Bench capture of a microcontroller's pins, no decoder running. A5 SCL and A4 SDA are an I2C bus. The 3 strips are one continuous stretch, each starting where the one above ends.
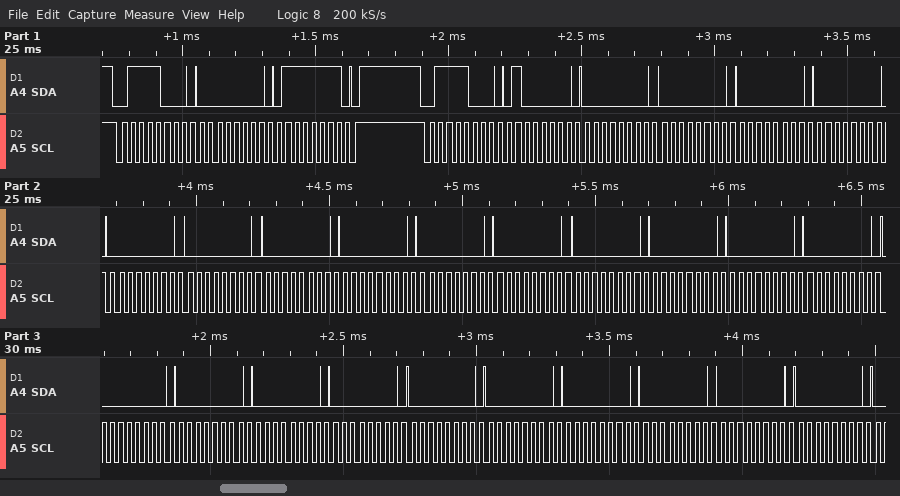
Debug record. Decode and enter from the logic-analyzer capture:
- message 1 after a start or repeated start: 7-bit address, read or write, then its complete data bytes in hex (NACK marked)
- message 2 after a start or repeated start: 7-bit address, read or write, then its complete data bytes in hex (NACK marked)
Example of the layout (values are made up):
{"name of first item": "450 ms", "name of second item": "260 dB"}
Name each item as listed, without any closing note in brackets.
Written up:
{"message 1 after a start or repeated start: 7-bit address, read or write, then its complete data bytes in hex": "0x3C write: 00 7F", "message 2 after a start or repeated start: 7-bit address, read or write, then its complete data bytes in hex": "0x3C write: 40 00 00 00 00 00 00 00 00 00 00 00 00 00 00 00 00 00 00 00 00 00 00 00 00"}
